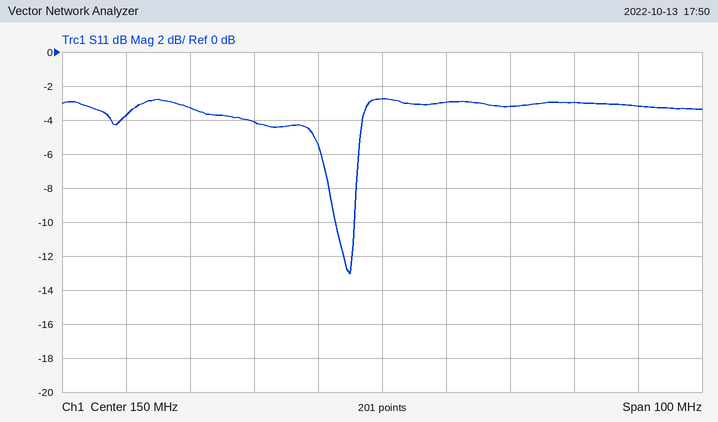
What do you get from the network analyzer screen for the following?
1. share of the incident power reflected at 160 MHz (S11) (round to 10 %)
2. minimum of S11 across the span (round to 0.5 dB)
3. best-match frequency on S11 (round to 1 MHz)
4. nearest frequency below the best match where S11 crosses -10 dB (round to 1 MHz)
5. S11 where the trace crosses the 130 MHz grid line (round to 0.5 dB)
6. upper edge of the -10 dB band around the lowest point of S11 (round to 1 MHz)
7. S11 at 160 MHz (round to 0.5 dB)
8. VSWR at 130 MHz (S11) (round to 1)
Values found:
50 %
-13.0 dB
145 MHz
143 MHz
-4.0 dB
146 MHz
-3.0 dB
4
